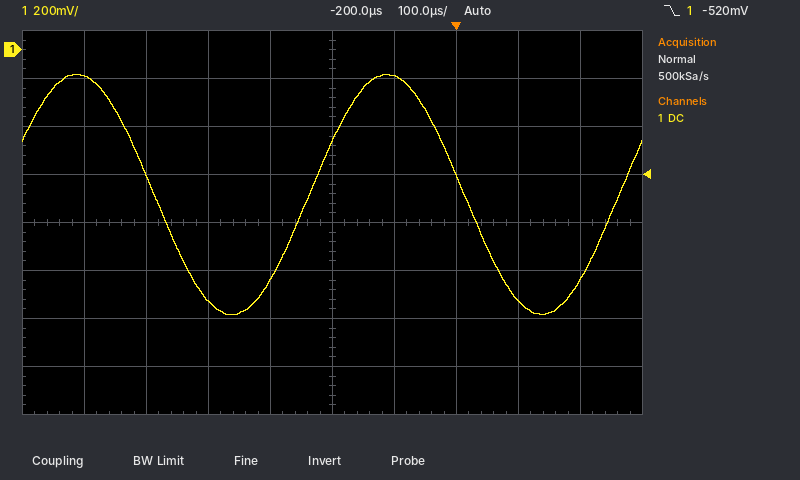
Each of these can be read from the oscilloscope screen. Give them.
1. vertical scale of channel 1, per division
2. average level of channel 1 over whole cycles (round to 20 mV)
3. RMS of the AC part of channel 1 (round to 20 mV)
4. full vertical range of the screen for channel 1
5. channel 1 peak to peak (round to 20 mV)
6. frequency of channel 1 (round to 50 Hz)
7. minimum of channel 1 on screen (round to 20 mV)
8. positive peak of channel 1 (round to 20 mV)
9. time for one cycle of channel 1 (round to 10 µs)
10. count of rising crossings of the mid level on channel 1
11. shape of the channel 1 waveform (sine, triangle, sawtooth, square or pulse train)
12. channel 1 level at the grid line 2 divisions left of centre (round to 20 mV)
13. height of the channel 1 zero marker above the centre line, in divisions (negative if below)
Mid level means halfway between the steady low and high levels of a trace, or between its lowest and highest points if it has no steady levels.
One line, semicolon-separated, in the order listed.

200 mV; -600 mV; 360 mV; 1.6 V; 1.00 V; 2.00 kHz; -1.10 V; -100 mV; 500 µs; 2; sine; -1.04 V; +3.6 div
